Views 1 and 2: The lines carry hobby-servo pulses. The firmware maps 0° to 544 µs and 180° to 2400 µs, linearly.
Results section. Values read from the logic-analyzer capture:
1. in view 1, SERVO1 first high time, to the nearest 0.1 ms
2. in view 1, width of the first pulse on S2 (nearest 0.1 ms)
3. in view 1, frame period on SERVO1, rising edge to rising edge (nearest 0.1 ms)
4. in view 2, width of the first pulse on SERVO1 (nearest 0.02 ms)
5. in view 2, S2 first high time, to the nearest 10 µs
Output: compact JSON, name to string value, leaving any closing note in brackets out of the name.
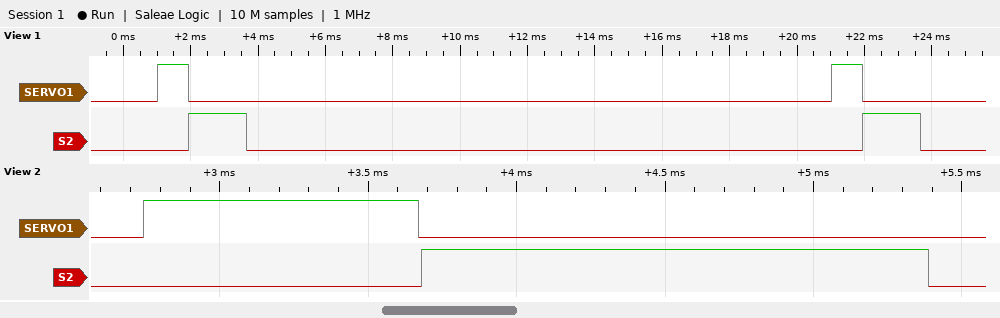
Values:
{"in view 1, SERVO1 first high time, to the nearest 0.1 ms": "0.9 ms", "in view 1, width of the first pulse on S2": "1.7 ms", "in view 1, frame period on SERVO1, rising edge to rising edge": "20.0 ms", "in view 2, width of the first pulse on SERVO1": "0.92 ms", "in view 2, S2 first high time, to the nearest 10 µs": "1710 µs"}
